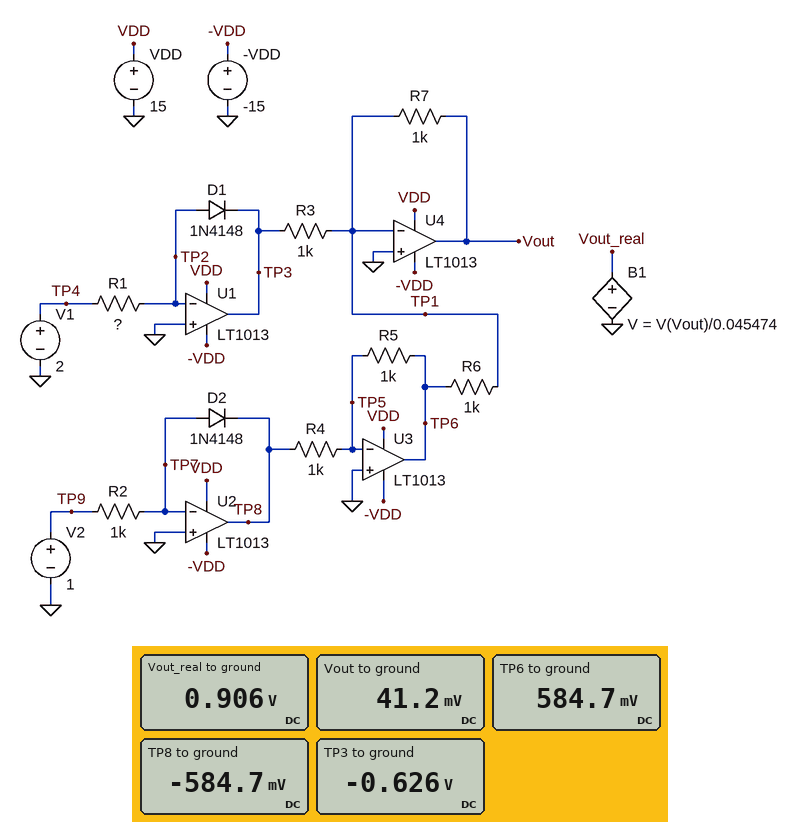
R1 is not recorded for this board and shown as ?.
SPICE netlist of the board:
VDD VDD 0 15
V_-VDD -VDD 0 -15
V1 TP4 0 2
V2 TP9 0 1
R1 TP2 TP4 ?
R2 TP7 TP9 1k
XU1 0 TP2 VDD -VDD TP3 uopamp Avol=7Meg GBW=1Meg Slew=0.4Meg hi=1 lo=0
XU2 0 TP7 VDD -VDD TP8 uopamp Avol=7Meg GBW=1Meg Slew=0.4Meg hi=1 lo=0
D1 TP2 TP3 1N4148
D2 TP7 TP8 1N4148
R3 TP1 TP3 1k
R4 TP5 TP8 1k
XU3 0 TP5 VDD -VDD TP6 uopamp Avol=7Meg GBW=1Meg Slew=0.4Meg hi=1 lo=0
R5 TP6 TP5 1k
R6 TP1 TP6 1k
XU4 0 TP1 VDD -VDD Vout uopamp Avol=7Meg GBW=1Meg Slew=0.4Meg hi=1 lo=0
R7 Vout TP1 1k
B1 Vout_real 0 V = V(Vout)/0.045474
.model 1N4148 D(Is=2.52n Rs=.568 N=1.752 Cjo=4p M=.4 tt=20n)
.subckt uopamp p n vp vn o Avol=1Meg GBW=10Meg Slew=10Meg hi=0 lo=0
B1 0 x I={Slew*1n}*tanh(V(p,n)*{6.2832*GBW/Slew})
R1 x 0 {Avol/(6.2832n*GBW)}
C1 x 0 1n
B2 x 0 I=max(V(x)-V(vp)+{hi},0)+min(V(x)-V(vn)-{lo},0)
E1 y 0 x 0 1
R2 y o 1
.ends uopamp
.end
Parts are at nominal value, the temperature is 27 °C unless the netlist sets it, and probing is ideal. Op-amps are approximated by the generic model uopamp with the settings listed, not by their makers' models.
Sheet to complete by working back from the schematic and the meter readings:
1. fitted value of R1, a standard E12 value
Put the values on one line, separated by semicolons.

820 Ω
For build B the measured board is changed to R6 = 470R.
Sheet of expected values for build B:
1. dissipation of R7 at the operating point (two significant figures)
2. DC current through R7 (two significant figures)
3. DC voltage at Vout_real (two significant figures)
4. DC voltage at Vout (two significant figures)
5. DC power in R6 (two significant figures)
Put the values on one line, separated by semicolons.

380 µW; 620 µA; -14 V; -620 mV; 730 µW
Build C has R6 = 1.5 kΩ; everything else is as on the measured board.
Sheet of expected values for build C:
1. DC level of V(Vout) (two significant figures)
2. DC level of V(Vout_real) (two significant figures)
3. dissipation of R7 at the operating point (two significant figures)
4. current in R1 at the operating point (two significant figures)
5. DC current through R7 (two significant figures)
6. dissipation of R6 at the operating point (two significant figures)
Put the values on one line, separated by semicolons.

240 mV; 5.2 V; 56 µW; 2.4 mA; 240 µA; 230 µW
